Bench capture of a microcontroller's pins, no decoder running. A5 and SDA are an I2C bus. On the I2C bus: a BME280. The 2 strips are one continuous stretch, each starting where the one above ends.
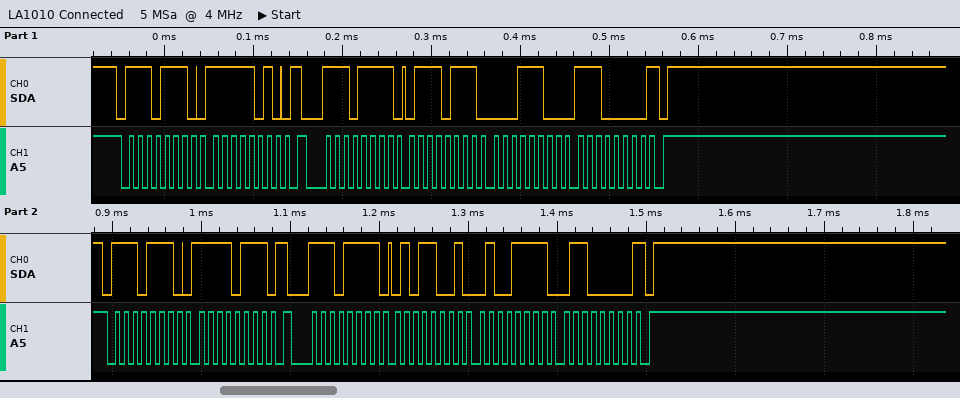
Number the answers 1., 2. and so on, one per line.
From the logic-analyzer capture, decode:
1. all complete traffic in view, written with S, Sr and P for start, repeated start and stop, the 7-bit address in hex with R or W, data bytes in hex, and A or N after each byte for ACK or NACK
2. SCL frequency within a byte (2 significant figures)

1. S 77W A FA A Sr 77R A 77 A 1C A E0 N P S 77W A F7 A Sr 77R A 59 A 4F A 60 N P
2. 100 kHz
